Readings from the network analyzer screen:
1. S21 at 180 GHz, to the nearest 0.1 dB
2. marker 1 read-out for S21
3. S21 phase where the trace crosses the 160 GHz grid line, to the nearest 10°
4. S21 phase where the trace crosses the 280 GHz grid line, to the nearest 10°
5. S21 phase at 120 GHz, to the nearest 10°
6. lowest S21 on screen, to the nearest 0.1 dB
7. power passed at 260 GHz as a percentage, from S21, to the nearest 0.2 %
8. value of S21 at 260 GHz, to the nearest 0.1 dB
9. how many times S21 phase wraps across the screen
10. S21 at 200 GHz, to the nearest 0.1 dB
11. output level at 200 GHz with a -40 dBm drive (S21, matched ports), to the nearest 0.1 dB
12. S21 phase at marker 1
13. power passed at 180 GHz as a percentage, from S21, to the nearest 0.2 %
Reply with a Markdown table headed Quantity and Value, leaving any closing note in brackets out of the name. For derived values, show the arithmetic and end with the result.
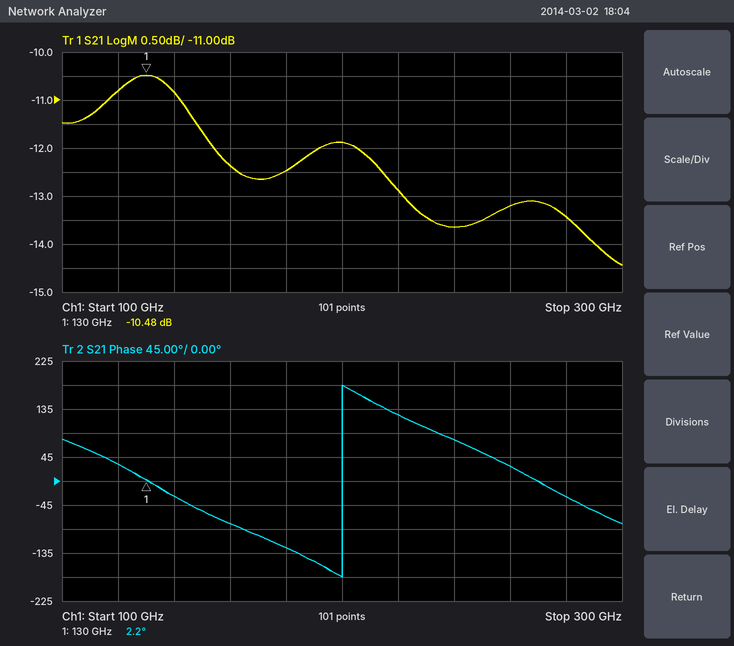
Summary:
| Quantity | Value |
|---|---|
| S21 at 180 GHz, to the nearest 0.1 dB | -12.5 dB |
| marker 1 read-out for S21 | -10.48 dB |
| S21 phase where the trace crosses the 160 GHz grid line, to the nearest 10° | -80° |
| S21 phase where the trace crosses the 280 GHz grid line, to the nearest 10° | -30° |
| S21 phase at 120 GHz, to the nearest 10° | 30° |
| lowest S21 on screen, to the nearest 0.1 dB | -14.4 dB |
| power passed at 260 GHz as a percentage, from S21, to the nearest 0.2 % | 10^(-13.2/10) ≈ 4.8 % |
| value of S21 at 260 GHz, to the nearest 0.1 dB | -13.2 dB |
| how many times S21 phase wraps across the screen | 1 |
| S21 at 200 GHz, to the nearest 0.1 dB | -11.9 dB |
| output level at 200 GHz with a -40 dBm drive (S21, matched ports), to the nearest 0.1 dB | -40 dBm + (-11.9 dB) = -51.9 dBm |
| S21 phase at marker 1 | 2.2° |
| power passed at 180 GHz as a percentage, from S21, to the nearest 0.2 % | 10^(-12.5/10) ≈ 5.6 % |
